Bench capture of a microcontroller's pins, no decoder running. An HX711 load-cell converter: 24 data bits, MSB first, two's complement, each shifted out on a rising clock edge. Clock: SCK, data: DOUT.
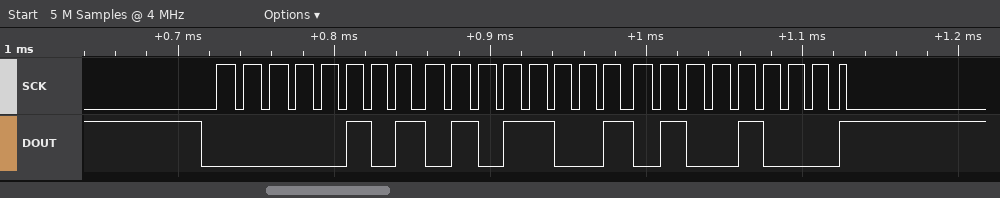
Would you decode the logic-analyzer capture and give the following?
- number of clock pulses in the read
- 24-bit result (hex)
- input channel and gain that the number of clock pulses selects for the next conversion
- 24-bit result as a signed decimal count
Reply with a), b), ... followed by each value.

a) 25
b) 0x055948
c) channel A, gain 128
d) 350536
